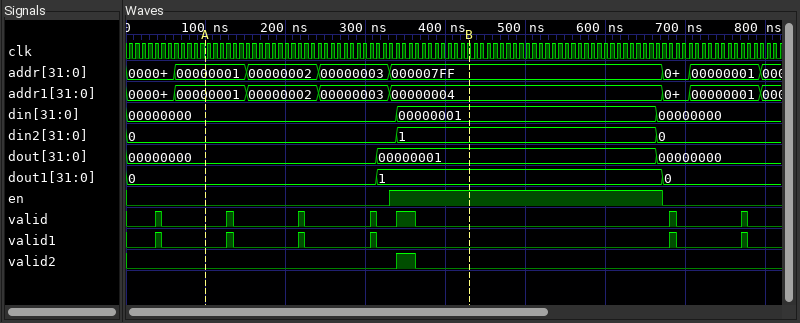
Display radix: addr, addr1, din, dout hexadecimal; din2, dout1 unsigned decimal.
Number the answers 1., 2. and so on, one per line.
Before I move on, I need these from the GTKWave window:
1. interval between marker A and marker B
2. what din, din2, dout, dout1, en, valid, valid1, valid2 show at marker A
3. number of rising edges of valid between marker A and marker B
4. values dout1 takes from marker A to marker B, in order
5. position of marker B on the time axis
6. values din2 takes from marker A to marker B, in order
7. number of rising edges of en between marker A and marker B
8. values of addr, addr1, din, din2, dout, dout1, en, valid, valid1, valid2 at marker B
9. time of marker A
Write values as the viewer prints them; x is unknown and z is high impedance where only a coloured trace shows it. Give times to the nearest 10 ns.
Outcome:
1. 330 ns
2. din=00000000, din2=0, dout=00000000, dout1=0, en=0, valid=0, valid1=0, valid2=0
3. 4
4. 0, 1
5. 430 ns
6. 0, 1
7. 1
8. addr=000007FF, addr1=00000004, din=00000001, din2=1, dout=00000001, dout1=1, en=1, valid=0, valid1=0, valid2=0
9. 100 ns
